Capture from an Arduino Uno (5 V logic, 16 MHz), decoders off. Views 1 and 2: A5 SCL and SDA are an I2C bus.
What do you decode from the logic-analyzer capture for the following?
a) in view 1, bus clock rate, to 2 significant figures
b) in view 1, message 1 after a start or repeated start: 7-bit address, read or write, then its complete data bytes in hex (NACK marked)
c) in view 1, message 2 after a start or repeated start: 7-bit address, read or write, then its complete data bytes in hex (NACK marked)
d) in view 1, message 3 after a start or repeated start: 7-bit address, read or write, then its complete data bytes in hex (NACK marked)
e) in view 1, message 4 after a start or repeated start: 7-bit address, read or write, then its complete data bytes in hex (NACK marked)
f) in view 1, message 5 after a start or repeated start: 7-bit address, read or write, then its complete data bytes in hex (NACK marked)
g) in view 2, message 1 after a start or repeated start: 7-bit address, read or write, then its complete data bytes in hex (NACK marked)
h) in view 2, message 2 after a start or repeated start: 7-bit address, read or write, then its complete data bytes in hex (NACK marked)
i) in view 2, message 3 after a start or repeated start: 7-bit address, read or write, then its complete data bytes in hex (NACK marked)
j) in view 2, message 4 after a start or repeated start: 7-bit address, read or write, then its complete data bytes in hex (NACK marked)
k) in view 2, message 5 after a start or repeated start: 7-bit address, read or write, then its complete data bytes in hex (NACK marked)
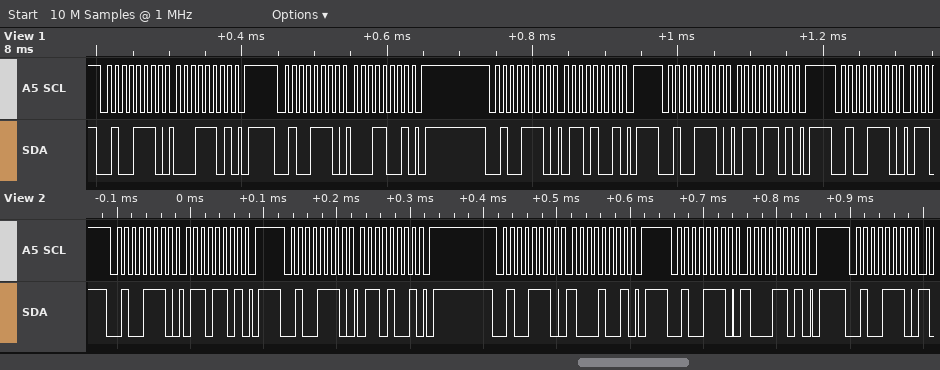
100 kHz
0x27 write: 1D
0x27 write: 19
0x27 write: 69
0x27 write: 6D
0x27 write
0x27 write: 6D
0x27 write: 69
0x27 write: 89
0x27 write: 8D
0x27 write
